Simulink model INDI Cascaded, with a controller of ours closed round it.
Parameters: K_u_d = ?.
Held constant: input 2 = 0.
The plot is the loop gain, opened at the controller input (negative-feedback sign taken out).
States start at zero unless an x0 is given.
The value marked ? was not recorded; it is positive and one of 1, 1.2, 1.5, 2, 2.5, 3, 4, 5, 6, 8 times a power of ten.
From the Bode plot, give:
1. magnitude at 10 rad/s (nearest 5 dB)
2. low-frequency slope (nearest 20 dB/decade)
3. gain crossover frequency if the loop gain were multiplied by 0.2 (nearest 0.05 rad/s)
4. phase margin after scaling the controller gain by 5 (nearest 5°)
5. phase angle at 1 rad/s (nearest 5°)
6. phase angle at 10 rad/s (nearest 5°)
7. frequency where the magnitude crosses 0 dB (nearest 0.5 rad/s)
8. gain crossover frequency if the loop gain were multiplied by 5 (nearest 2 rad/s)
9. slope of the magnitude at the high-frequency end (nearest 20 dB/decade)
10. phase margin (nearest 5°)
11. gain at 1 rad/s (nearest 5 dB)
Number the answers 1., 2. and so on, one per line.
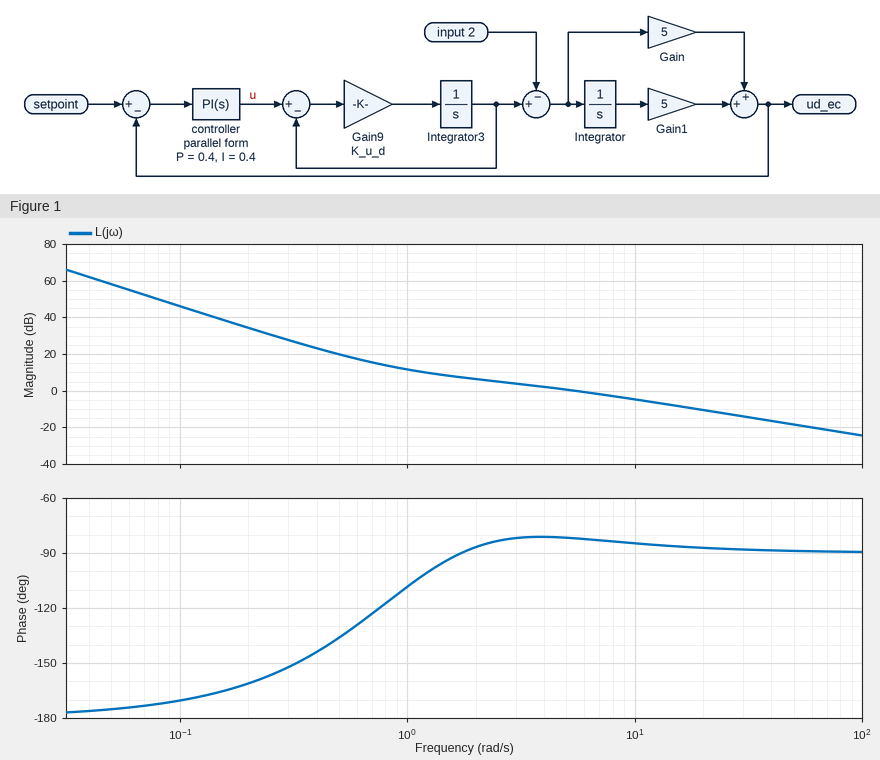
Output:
1. -5 dB
2. -40 dB/decade
3. 0.80 rad/s
4. 90°
5. -110°
6. -85°
7. 5.5 rad/s
8. 30 rad/s
9. -20 dB/decade
10. 100°
11. 10 dB
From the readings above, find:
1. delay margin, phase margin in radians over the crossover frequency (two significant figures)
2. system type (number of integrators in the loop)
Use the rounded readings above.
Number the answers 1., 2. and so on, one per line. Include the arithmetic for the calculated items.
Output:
1. 100 × π / 180 / 5.5 = 0.32 s
2. 2
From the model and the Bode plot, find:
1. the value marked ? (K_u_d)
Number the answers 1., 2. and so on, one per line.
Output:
1. 3
